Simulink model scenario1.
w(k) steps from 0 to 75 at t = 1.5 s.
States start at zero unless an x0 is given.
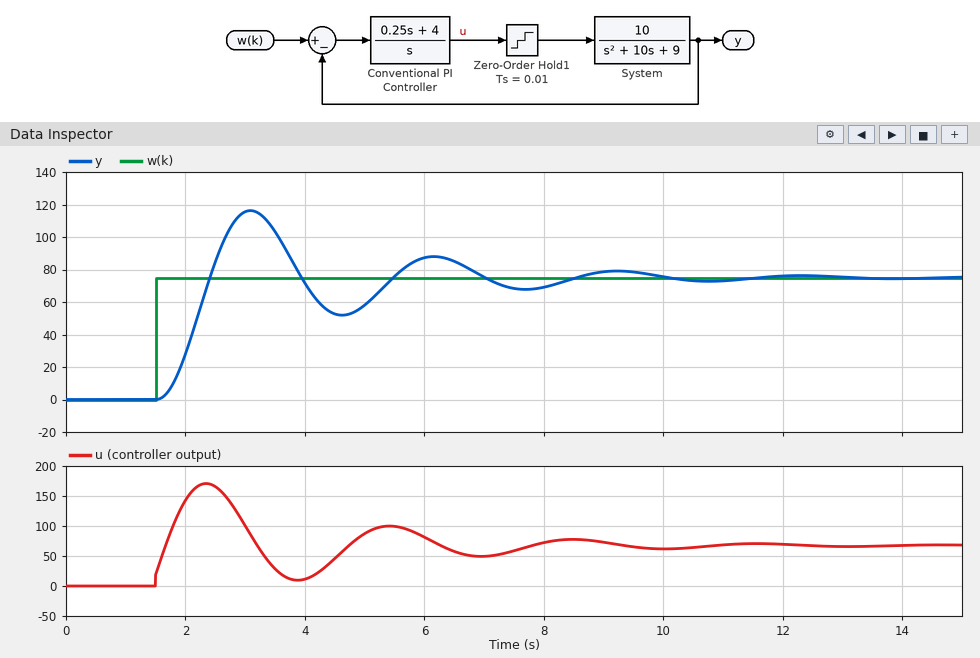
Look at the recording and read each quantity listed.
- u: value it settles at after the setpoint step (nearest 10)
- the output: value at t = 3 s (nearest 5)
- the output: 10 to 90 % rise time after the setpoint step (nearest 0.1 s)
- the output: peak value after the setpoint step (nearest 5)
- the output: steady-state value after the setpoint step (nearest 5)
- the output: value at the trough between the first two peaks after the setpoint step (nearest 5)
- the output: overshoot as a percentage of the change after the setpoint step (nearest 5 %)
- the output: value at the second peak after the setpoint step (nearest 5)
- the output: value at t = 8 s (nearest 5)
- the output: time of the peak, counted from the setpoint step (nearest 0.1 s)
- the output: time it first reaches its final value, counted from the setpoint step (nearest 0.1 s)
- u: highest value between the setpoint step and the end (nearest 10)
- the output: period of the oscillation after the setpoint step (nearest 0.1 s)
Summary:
70
115
0.6 s
115
75
50
55 %
90
70
1.6 s
0.9 s
170
3.1 s
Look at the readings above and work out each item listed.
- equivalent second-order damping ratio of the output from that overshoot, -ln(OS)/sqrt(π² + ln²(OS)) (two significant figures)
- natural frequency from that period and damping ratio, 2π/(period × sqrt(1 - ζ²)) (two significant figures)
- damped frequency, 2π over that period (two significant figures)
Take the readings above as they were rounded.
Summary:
0.19
2.1 rad/s
2.0 rad/s
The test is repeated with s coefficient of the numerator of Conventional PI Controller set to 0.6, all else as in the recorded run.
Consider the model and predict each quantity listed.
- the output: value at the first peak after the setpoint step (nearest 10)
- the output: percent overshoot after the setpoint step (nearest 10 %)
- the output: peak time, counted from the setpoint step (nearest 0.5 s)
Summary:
110
40 %
1.5 s
